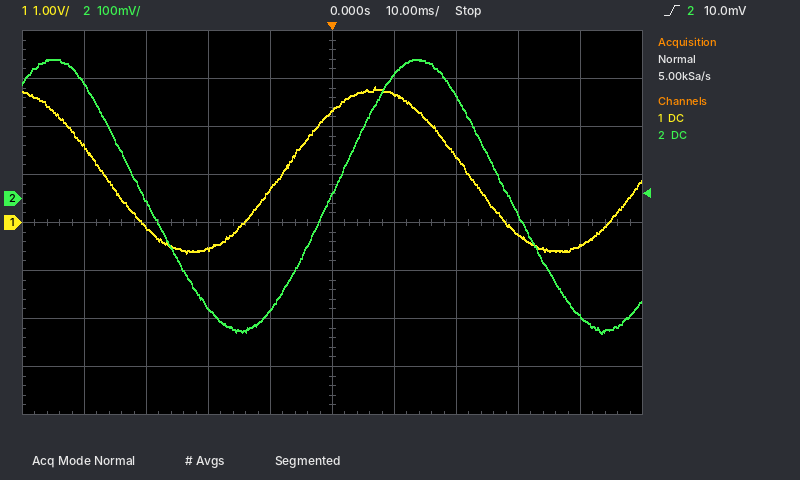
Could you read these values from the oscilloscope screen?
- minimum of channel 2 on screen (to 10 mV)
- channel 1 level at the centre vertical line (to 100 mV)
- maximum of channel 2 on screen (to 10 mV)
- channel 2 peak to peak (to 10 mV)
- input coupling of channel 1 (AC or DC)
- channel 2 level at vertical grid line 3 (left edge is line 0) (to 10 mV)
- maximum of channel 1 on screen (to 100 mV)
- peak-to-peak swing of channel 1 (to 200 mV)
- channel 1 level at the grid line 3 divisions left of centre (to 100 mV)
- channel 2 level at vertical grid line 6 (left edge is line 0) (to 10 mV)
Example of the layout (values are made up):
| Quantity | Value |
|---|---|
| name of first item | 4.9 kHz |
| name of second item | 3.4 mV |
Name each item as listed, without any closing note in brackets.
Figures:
| Quantity | Value |
|---|---|
| minimum of channel 2 on screen | -280 mV |
| channel 1 level at the centre vertical line | 2.3 V |
| maximum of channel 2 on screen | 290 mV |
| channel 2 peak to peak | 570 mV |
| input coupling of channel 1 | DC |
| channel 2 level at vertical grid line 3 (left edge is line 0) | -230 mV |
| maximum of channel 1 on screen | 2.8 V |
| peak-to-peak swing of channel 1 | 3.4 V |
| channel 1 level at the grid line 3 divisions left of centre | -100 mV |
| channel 2 level at vertical grid line 6 (left edge is line 0) | 260 mV |
